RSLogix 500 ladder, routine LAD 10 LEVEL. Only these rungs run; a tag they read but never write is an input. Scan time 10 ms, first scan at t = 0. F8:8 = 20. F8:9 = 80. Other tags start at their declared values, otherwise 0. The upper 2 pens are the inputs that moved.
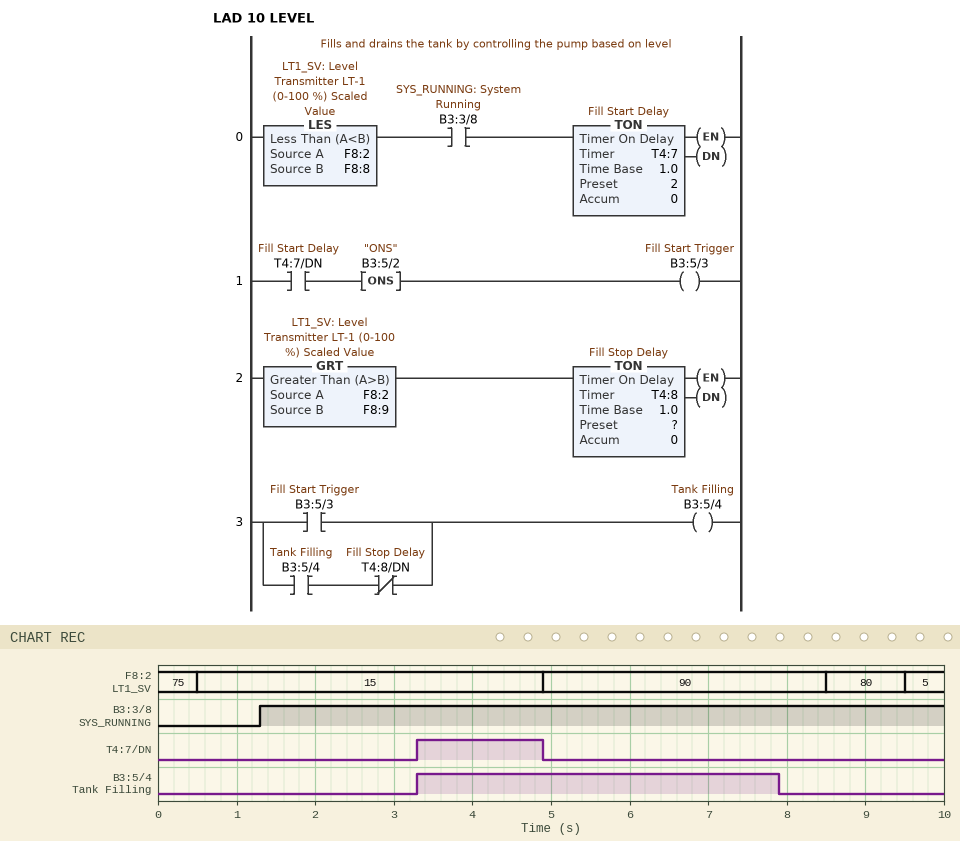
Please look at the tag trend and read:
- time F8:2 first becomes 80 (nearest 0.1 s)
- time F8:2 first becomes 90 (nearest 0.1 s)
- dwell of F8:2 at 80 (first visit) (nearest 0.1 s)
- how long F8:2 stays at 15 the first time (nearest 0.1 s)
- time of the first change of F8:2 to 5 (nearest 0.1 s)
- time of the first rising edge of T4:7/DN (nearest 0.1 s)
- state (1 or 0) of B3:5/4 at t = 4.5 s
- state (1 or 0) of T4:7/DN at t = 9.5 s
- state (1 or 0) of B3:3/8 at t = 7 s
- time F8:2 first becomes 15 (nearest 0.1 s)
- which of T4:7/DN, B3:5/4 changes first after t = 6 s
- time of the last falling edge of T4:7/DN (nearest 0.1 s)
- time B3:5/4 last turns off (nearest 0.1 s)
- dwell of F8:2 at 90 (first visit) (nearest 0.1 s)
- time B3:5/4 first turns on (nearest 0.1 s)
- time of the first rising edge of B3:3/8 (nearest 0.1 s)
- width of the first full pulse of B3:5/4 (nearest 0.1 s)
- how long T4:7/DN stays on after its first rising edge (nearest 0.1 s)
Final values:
8.5 s
4.9 s
1.0 s
4.4 s
9.5 s
3.3 s
1
0
1
0.5 s
B3:5/4
4.9 s
7.9 s
3.6 s
3.3 s
1.3 s
4.6 s
1.6 s
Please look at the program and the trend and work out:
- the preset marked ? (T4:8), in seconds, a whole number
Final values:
3 s
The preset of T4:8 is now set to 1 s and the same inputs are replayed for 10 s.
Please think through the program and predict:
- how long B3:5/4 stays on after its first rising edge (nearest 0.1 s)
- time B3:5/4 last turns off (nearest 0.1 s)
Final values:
2.6 s
5.9 s
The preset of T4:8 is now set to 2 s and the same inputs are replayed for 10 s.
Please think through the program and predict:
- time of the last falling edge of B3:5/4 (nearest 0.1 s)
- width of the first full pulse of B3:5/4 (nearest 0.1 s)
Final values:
6.9 s
3.6 s
